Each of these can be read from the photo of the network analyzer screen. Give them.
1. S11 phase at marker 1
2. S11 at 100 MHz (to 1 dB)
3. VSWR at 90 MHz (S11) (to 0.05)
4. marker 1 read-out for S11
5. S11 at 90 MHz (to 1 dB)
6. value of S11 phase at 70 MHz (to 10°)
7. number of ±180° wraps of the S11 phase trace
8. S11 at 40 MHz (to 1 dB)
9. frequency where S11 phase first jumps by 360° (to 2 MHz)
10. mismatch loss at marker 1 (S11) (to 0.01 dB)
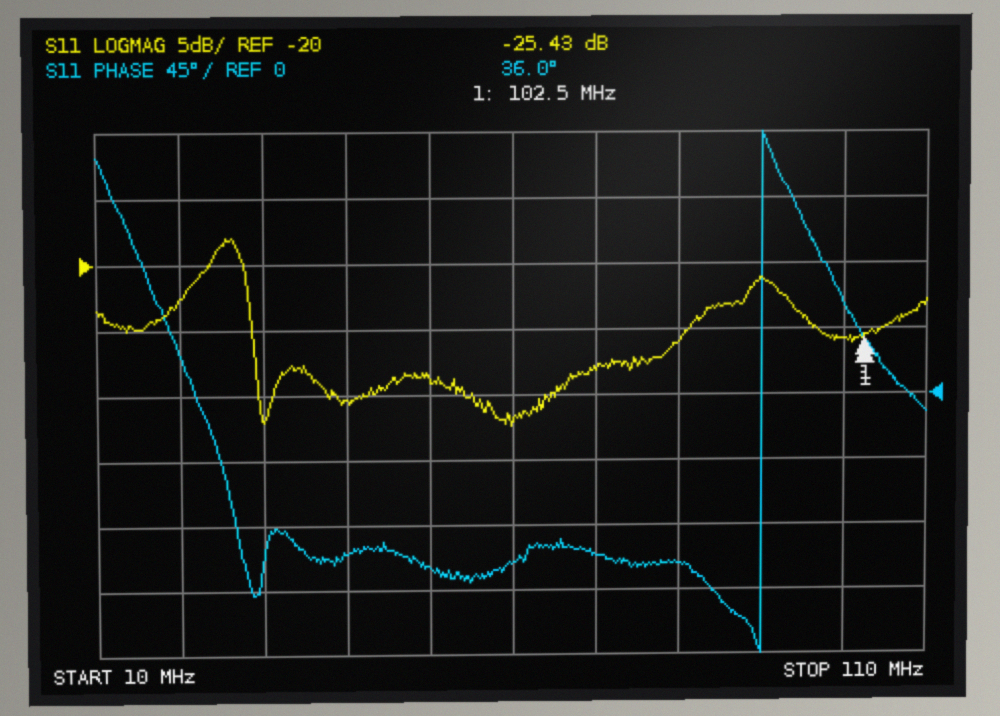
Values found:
36.0°
-26 dB
1.20
-25.43 dB
-21 dB
-110°
1
-30 dB
90 MHz
0.01 dB
